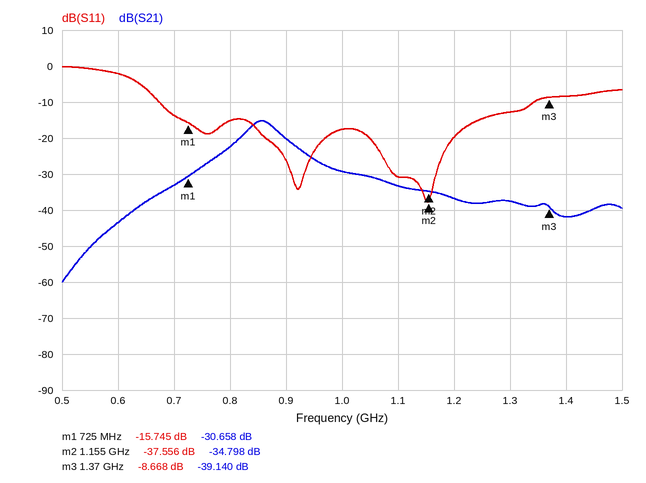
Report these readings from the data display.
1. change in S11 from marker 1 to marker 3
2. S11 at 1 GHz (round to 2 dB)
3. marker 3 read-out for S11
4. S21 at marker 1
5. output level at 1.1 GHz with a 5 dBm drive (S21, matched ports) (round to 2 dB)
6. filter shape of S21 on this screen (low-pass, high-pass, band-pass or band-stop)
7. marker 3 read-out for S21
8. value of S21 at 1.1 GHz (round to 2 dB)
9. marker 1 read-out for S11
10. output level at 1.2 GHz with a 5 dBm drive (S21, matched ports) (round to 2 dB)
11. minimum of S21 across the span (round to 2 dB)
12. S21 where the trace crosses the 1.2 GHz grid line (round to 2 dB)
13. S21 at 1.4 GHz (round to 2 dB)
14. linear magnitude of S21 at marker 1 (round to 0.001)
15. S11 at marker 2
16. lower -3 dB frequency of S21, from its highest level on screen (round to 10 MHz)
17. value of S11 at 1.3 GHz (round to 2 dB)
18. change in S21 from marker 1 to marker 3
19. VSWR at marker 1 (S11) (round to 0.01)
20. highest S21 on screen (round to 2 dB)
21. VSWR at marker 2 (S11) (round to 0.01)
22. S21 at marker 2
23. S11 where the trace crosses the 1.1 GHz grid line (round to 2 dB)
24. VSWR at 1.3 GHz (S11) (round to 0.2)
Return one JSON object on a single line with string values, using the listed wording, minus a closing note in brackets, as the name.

{"change in S11 from marker 1 to marker 3": "7.077 dB", "S11 at 1 GHz": "-18 dB", "marker 3 read-out for S11": "-8.668 dB", "S21 at marker 1": "-30.658 dB", "output level at 1.1 GHz with a 5 dBm drive (S21, matched ports)": "-28 dBm", "filter shape of S21 on this screen": "band-pass", "marker 3 read-out for S21": "-39.140 dB", "value of S21 at 1.1 GHz": "-34 dB", "marker 1 read-out for S11": "-15.745 dB", "output level at 1.2 GHz with a 5 dBm drive (S21, matched ports)": "-32 dBm", "minimum of S21 across the span": "-60 dB", "S21 where the trace crosses the 1.2 GHz grid line": "-36 dB", "S21 at 1.4 GHz": "-42 dB", "linear magnitude of S21 at marker 1": "0.029", "S11 at marker 2": "-37.556 dB", "lower -3 dB frequency of S21, from its highest level on screen": "830 MHz", "value of S11 at 1.3 GHz": "-12 dB", "change in S21 from marker 1 to marker 3": "-8.482 dB", "VSWR at marker 1 (S11)": "1.39", "highest S21 on screen": "-16 dB", "VSWR at marker 2 (S11)": "1.03", "S21 at marker 2": "-34.798 dB", "S11 where the trace crosses the 1.1 GHz grid line": "-30 dB", "VSWR at 1.3 GHz (S11)": "1.6"}
